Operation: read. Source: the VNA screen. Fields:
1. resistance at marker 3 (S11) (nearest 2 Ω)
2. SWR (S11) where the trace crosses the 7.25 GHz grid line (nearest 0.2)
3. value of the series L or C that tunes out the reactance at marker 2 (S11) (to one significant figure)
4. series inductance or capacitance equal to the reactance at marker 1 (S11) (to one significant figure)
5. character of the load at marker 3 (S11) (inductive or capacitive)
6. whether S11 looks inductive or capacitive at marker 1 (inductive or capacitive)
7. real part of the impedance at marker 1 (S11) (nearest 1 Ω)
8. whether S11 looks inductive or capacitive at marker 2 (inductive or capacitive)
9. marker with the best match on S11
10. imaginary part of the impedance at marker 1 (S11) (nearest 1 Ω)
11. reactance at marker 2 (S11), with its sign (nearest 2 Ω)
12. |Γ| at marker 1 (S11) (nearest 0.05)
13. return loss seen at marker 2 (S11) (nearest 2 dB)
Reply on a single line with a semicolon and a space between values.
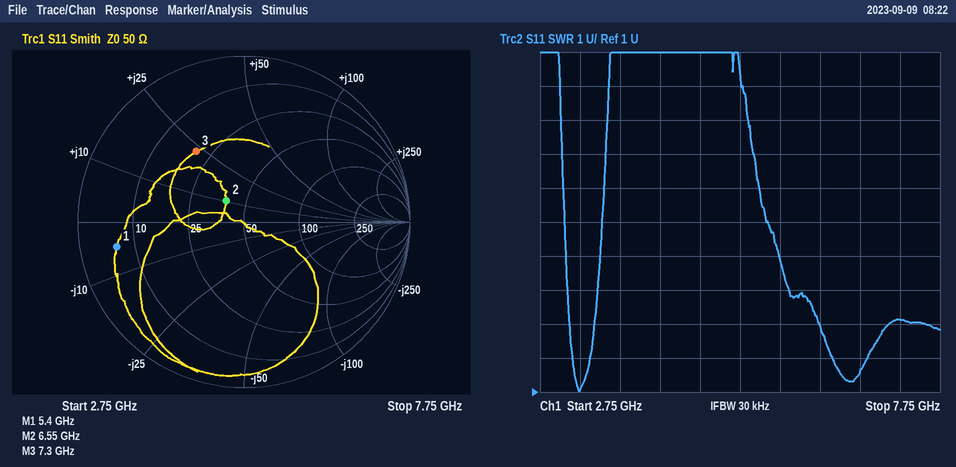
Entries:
20 Ω; 3.2; 2 pF; 6 pF; inductive; capacitive; 6 Ω; inductive; marker 2; -5 Ω; +10 Ω; 0.80; 16 dB
